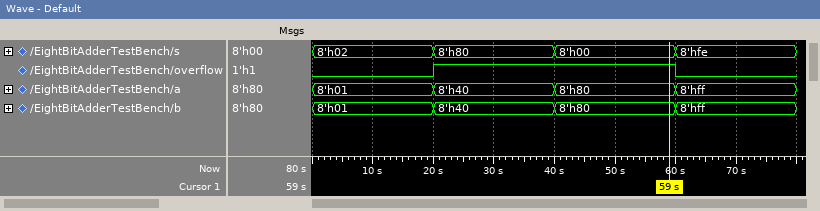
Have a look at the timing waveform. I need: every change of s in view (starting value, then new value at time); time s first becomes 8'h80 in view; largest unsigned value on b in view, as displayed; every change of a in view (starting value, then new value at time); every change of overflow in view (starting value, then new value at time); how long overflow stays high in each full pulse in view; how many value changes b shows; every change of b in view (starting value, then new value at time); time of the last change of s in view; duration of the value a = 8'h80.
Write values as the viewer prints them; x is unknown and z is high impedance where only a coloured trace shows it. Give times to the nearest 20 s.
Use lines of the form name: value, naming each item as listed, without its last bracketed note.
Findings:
every change of s in view: 8'h02, 8'h80 at 20 s, 8'h00 at 40 s, 8'hfe at 60 s
time s first becomes 8'h80 in view: 20 s
largest unsigned value on b in view, as displayed: 8'hff
every change of a in view: 8'h01, 8'h40 at 20 s, 8'h80 at 40 s, 8'hff at 60 s
every change of overflow in view: 0, 1 at 20 s, 0 at 60 s
how long overflow stays high in each full pulse in view: 40 s
how many value changes b shows: 3
every change of b in view: 8'h01, 8'h40 at 20 s, 8'h80 at 40 s, 8'hff at 60 s
time of the last change of s in view: 60 s
duration of the value a = 8'h80: 20 s
